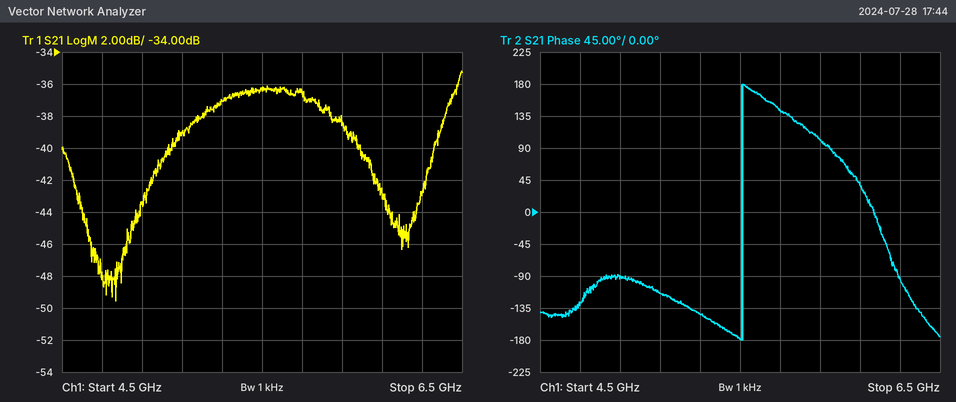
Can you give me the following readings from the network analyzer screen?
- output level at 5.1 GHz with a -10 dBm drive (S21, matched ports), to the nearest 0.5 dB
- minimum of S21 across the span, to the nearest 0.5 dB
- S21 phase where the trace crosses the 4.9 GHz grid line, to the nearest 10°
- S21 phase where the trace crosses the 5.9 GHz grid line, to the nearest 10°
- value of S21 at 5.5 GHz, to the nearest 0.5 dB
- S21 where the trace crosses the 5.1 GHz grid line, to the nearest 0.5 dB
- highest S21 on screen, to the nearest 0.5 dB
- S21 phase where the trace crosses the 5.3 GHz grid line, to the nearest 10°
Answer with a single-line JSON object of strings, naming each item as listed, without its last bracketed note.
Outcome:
{"output level at 5.1 GHz with a -10 dBm drive (S21, matched ports), to the nearest 0.5 dB": "-49.0 dBm", "minimum of S21 across the span, to the nearest 0.5 dB": "-49.5 dB", "S21 phase where the trace crosses the 4.9 GHz grid line, to the nearest 10°": "-90°", "S21 phase where the trace crosses the 5.9 GHz grid line, to the nearest 10°": "100°", "value of S21 at 5.5 GHz, to the nearest 0.5 dB": "-36.5 dB", "S21 where the trace crosses the 5.1 GHz grid line, to the nearest 0.5 dB": "-39.0 dB", "highest S21 on screen, to the nearest 0.5 dB": "-35.0 dB", "S21 phase where the trace crosses the 5.3 GHz grid line, to the nearest 10°": "-140°"}
